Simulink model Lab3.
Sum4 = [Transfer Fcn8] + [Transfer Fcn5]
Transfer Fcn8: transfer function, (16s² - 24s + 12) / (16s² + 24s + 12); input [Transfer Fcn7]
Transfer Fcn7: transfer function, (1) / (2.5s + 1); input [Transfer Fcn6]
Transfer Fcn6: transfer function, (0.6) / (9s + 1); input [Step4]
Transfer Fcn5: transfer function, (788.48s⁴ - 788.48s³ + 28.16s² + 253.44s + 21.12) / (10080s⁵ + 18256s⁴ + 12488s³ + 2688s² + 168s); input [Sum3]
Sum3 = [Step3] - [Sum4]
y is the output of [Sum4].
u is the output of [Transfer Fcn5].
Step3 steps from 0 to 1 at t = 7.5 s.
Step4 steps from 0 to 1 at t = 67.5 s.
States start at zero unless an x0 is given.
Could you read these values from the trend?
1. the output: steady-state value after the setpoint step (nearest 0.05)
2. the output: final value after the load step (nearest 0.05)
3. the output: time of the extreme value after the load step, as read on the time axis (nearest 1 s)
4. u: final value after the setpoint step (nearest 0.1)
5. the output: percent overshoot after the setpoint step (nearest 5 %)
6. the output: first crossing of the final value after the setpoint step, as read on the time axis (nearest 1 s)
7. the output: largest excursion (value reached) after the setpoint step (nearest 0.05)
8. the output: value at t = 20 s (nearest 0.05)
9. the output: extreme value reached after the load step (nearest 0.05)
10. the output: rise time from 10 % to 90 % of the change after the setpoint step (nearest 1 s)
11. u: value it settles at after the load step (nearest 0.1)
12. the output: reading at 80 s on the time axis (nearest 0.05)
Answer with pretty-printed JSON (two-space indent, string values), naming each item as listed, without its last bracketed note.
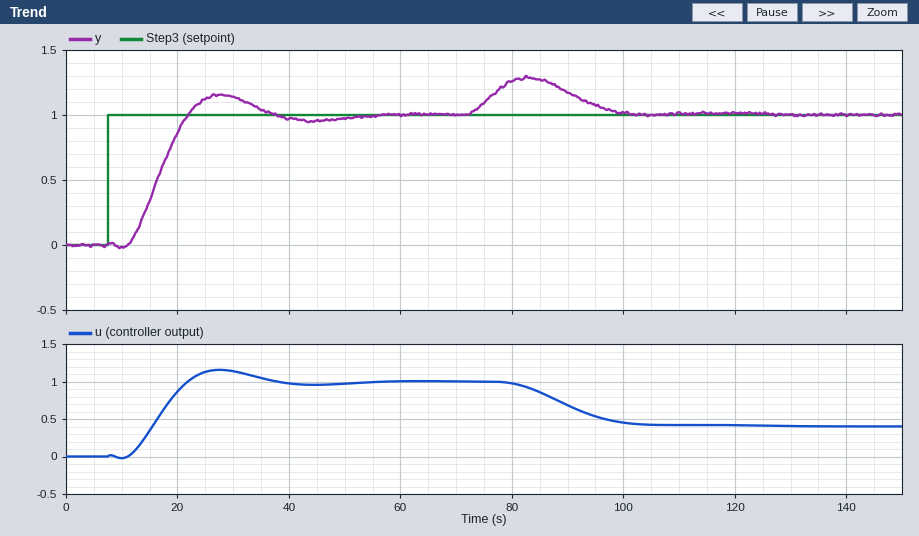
{
  "the output: steady-state value after the setpoint step": "1.00",
  "the output: final value after the load step": "1.00",
  "the output: time of the extreme value after the load step, as read on the time axis": "83 s",
  "u: final value after the setpoint step": "1.0",
  "the output: percent overshoot after the setpoint step": "15 %",
  "the output: first crossing of the final value after the setpoint step, as read on the time axis": "22 s",
  "the output: largest excursion (value reached) after the setpoint step": "1.15",
  "the output: value at t = 20 s": "0.85",
  "the output: extreme value reached after the load step": "1.30",
  "the output: rise time from 10 % to 90 % of the change after the setpoint step": "8 s",
  "u: value it settles at after the load step": "0.4",
  "the output: reading at 80 s on the time axis": "1.25"
}
